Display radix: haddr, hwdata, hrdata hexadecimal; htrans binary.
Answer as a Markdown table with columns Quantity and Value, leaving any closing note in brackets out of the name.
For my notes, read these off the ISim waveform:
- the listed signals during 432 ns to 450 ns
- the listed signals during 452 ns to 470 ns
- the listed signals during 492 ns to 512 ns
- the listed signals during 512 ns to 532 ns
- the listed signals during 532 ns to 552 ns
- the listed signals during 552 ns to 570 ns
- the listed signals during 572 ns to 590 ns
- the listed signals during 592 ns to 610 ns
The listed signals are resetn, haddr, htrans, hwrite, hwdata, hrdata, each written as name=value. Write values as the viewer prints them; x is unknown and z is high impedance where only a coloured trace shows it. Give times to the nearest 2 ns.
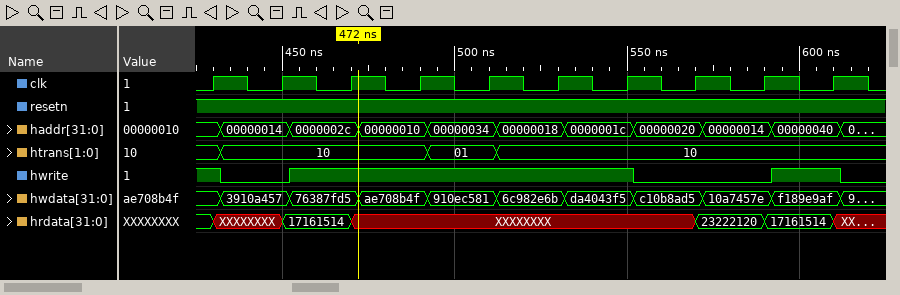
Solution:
| Quantity | Value |
|---|---|
| the listed signals during 432 ns to 450 ns | resetn=1, haddr=00000014, htrans=10, hwrite=0, hwdata=3910a457, hrdata=XXXXXXXX |
| the listed signals during 452 ns to 470 ns | resetn=1, haddr=0000002c, htrans=10, hwrite=1, hwdata=76387fd5, hrdata=17161514 |
| the listed signals during 492 ns to 512 ns | resetn=1, haddr=00000034, htrans=01, hwrite=1, hwdata=910ec581, hrdata=XXXXXXXX |
| the listed signals during 512 ns to 532 ns | resetn=1, haddr=00000018, htrans=10, hwrite=1, hwdata=6c982e6b, hrdata=XXXXXXXX |
| the listed signals during 532 ns to 552 ns | resetn=1, haddr=0000001c, htrans=10, hwrite=1, hwdata=da4043f5, hrdata=XXXXXXXX |
| the listed signals during 552 ns to 570 ns | resetn=1, haddr=00000020, htrans=10, hwrite=0, hwdata=c10b8ad5, hrdata=XXXXXXXX |
| the listed signals during 572 ns to 590 ns | resetn=1, haddr=00000014, htrans=10, hwrite=0, hwdata=10a7457e, hrdata=23222120 |
| the listed signals during 592 ns to 610 ns | resetn=1, haddr=00000040, htrans=10, hwrite=1, hwdata=f189e9af, hrdata=17161514 |
